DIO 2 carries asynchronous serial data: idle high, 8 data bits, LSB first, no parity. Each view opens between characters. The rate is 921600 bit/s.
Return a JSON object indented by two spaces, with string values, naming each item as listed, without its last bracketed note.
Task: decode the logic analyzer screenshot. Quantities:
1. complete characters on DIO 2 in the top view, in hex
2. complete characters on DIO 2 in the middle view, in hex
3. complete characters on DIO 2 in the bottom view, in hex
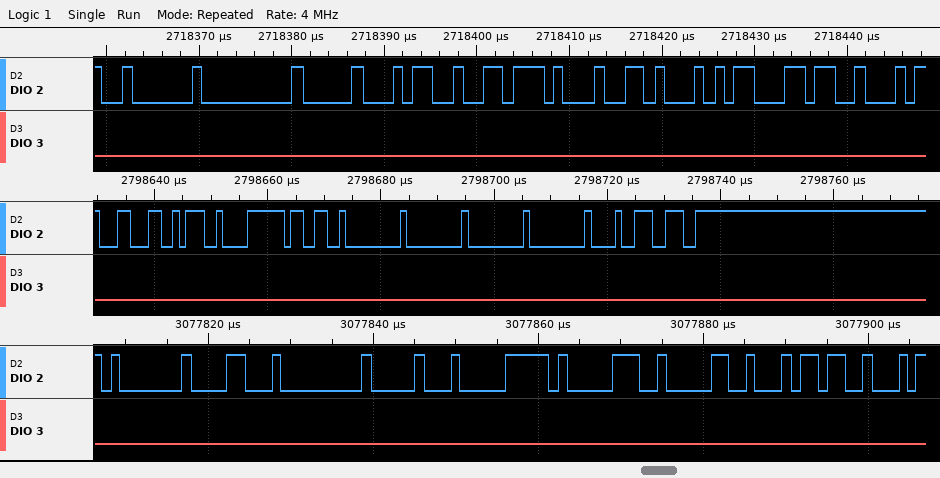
{
  "complete characters on DIO 2 in the top view, in hex": "02, 00, 10, 93, 17, 16, 8D, 13",
  "complete characters on DIO 2 in the middle view, in hex": "8C, 3A, F8, 33, 00, 00, 00, 00, C8, CE",
  "complete characters on DIO 2 in the bottom view, in hex": "01, 18, 00, 10, F0, C1, 82, A2, 13"
}
